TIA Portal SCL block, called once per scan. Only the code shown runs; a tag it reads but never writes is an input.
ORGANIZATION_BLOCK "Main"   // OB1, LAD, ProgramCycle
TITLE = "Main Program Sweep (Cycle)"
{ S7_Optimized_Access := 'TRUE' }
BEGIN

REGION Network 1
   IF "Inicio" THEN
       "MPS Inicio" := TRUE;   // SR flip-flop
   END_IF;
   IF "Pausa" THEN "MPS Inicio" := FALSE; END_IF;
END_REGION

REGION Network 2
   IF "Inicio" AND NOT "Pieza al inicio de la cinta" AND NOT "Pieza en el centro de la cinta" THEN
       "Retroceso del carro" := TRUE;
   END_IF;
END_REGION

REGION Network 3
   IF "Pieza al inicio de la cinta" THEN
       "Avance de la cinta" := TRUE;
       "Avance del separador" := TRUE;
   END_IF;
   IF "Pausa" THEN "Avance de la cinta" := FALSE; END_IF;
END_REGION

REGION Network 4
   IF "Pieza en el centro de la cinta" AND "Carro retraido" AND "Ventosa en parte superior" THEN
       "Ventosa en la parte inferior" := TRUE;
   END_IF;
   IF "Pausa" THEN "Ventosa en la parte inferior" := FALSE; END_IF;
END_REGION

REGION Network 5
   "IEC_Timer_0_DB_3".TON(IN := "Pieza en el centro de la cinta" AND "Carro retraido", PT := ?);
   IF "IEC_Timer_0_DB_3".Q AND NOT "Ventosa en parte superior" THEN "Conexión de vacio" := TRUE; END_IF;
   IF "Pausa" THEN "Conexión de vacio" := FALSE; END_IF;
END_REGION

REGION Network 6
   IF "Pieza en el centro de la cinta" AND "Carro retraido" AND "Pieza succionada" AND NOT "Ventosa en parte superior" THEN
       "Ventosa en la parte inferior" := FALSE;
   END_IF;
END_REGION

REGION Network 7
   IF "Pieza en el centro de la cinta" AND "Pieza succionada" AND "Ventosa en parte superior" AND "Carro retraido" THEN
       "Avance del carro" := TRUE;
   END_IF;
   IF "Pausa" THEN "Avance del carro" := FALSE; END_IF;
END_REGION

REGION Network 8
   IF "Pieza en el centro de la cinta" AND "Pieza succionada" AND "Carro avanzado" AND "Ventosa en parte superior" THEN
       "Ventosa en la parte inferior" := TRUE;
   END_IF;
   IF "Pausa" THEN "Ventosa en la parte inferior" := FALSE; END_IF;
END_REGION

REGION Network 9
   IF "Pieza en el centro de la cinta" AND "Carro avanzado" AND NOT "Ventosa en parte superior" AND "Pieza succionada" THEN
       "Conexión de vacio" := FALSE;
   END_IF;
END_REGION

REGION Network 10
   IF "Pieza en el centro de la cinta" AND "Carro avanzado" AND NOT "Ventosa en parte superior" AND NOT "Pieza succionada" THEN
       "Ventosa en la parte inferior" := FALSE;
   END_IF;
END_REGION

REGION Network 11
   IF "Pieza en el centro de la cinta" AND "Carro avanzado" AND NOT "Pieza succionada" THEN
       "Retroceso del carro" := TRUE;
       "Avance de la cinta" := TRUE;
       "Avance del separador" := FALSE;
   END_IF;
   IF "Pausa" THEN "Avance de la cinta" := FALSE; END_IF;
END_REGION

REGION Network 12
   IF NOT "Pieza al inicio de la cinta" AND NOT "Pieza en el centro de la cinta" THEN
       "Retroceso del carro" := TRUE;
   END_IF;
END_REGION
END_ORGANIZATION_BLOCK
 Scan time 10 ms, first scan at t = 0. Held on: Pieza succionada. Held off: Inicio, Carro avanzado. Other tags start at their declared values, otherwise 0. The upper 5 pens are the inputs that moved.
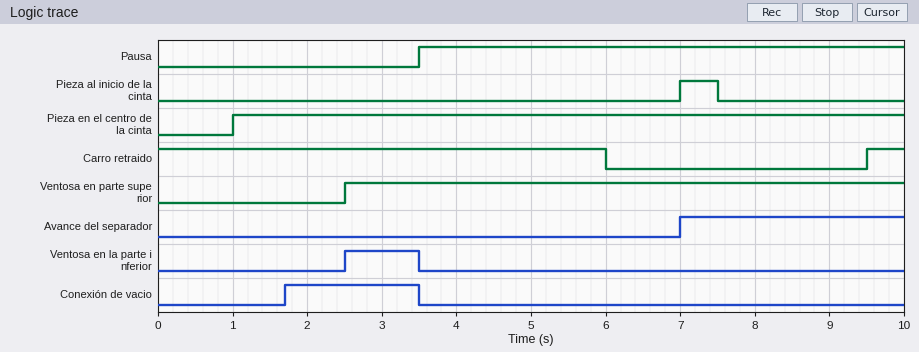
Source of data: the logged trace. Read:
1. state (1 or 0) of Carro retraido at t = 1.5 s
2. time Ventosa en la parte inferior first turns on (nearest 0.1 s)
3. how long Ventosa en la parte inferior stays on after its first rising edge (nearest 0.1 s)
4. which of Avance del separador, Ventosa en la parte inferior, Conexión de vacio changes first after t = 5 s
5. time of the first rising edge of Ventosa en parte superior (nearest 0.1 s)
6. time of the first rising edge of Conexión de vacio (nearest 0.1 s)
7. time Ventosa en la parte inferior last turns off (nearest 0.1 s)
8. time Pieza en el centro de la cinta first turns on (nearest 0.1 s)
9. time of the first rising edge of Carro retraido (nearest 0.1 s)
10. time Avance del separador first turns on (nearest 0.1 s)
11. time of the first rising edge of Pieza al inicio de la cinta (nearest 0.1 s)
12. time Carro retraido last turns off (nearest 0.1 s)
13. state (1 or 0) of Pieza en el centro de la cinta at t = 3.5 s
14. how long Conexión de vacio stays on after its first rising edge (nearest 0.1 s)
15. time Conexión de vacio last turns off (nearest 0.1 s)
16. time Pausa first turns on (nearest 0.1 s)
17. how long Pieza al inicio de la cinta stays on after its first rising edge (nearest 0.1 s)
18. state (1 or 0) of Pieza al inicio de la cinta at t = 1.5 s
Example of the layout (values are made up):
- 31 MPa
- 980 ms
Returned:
- 1
- 2.5 s
- 1.0 s
- Avance del separador
- 2.5 s
- 1.7 s
- 3.5 s
- 1.0 s
- 9.5 s
- 7.0 s
- 7.0 s
- 6.0 s
- 1
- 1.8 s
- 3.5 s
- 3.5 s
- 0.5 s
- 0
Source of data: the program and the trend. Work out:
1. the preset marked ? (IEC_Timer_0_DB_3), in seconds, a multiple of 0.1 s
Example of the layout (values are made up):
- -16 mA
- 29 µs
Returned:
- 0.7 s
